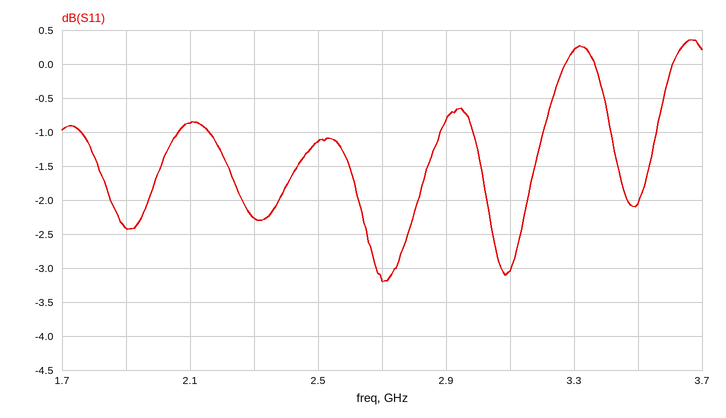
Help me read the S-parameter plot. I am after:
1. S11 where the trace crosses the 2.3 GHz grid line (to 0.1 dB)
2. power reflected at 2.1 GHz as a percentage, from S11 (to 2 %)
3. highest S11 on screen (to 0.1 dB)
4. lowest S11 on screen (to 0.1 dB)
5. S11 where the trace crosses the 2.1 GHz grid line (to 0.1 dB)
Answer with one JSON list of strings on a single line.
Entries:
["-2.3 dB", "82 %", "0.4 dB", "-3.2 dB", "-0.9 dB"]
